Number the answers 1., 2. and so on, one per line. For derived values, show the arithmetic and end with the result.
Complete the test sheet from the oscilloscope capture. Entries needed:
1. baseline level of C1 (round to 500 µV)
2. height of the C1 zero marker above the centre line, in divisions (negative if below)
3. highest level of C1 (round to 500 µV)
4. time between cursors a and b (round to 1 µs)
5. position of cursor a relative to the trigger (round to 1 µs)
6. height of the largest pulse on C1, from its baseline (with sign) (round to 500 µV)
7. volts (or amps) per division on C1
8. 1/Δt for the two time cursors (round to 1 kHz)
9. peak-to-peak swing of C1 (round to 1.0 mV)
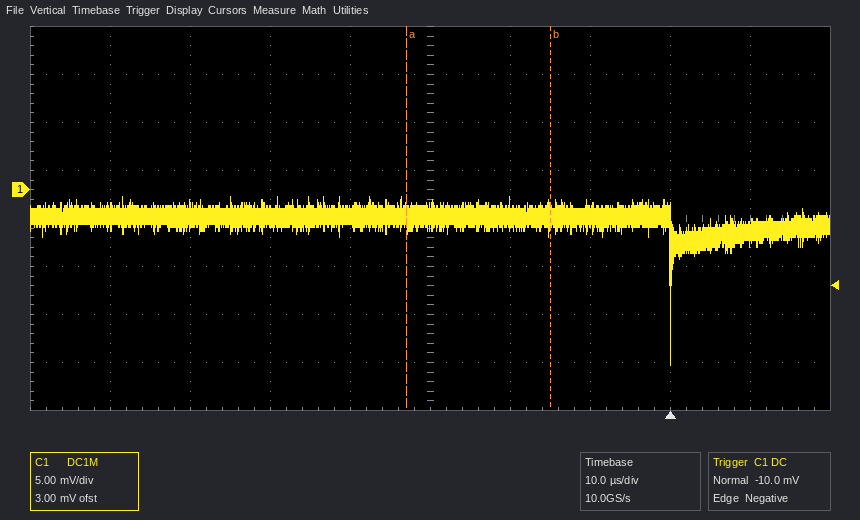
1. -3.0 mV
2. +0.6 div
3. -500 µV
4. 18 µs
5. -33 µs
6. -15.5 mV
7. 5 mV
8. 1 / 18 µs ≈ 56 kHz
9. 18.0 mV
